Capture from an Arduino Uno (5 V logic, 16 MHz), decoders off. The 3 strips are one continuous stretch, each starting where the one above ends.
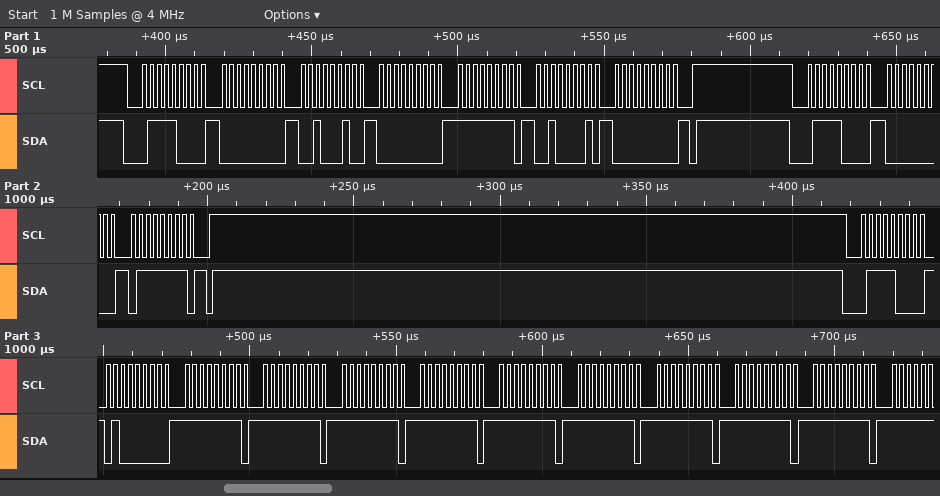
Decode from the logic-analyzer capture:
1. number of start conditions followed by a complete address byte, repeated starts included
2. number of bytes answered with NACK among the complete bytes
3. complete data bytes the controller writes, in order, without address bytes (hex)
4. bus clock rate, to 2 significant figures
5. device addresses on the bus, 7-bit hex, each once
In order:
3
0
00 22 00 FF 21 00 00 7F 40 FF FF FF FF FF FF FF FF FF
400 kHz
0x3C
